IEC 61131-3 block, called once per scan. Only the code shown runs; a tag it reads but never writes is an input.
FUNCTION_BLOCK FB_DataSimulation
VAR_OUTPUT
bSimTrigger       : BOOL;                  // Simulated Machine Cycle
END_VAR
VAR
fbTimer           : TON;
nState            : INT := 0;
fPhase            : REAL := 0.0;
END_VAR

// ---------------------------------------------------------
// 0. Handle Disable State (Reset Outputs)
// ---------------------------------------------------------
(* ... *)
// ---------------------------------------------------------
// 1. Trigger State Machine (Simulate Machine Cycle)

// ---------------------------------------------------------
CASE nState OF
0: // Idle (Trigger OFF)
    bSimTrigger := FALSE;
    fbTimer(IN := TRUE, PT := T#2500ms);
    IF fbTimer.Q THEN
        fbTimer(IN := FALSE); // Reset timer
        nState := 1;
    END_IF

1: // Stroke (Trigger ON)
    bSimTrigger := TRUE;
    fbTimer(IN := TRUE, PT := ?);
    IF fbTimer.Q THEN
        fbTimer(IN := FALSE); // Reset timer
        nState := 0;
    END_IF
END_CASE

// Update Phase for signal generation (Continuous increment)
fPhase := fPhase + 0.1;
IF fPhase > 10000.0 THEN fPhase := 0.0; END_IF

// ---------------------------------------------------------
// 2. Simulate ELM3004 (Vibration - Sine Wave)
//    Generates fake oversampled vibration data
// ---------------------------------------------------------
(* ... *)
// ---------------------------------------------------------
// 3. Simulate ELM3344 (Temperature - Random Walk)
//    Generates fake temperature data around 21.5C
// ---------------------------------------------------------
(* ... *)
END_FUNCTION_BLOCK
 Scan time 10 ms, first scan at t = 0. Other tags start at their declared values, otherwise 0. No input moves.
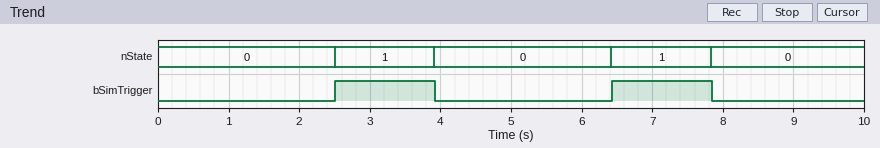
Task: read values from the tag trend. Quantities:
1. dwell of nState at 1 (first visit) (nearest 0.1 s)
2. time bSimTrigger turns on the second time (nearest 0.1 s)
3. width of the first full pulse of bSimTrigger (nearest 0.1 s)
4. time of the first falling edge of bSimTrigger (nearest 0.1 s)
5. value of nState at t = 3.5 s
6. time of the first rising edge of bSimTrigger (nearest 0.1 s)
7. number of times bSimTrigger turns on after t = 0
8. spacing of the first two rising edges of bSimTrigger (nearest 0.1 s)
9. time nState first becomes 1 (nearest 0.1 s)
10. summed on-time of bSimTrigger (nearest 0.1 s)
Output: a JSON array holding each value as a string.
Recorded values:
["1.4 s", "6.4 s", "1.4 s", "3.9 s", "1", "2.5 s", "2", "3.9 s", "2.5 s", "2.8 s"]
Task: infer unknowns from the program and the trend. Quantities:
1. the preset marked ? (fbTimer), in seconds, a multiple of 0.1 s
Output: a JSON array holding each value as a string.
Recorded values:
["1.4 s"]
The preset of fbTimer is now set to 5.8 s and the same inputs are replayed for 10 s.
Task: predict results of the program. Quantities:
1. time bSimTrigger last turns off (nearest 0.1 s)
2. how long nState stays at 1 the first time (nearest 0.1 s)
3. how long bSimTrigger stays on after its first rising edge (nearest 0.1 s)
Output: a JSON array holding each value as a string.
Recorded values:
["8.3 s", "5.8 s", "5.8 s"]
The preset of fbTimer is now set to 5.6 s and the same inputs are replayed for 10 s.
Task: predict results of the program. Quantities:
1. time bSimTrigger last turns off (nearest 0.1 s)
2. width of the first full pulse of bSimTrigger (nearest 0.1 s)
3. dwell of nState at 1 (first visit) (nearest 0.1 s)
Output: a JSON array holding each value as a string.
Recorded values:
["8.1 s", "5.6 s", "5.6 s"]
